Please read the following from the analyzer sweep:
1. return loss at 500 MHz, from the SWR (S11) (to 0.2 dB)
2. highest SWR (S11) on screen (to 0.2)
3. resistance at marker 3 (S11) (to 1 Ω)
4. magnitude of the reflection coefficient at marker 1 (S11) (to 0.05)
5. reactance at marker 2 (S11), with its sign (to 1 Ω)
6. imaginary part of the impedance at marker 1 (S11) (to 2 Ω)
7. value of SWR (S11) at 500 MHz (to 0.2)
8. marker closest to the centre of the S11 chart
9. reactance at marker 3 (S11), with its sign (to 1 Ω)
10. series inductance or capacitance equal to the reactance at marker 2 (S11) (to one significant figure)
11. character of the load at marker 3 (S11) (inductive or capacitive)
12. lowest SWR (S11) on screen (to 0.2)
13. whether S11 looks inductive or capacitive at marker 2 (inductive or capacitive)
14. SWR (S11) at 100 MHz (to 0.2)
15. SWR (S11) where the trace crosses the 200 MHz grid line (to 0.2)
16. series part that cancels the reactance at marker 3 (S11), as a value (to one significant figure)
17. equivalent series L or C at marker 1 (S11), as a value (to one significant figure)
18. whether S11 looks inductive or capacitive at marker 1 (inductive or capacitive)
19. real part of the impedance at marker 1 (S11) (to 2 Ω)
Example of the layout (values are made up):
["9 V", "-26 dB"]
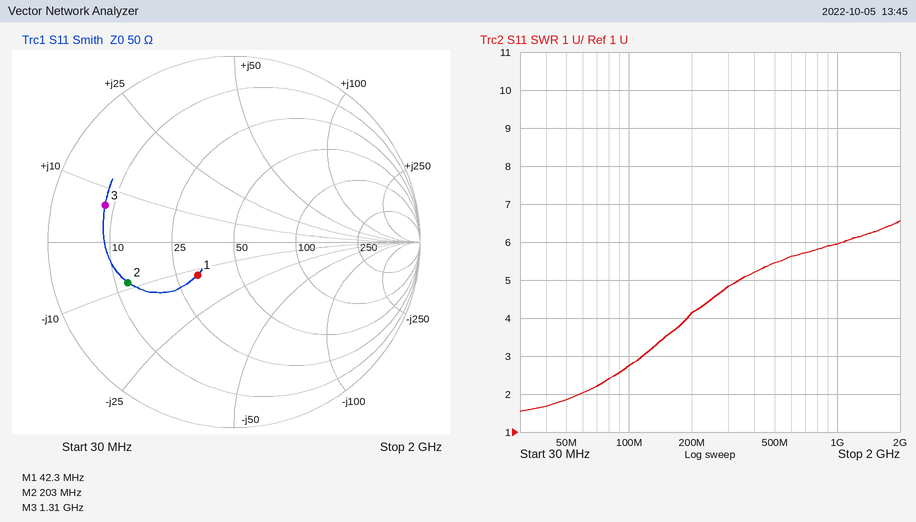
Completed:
["3.2 dB", "6.6", "8 Ω", "0.25", "-9 Ω", "-12 Ω", "5.4", "marker 1", "+7 Ω", "90 pF", "inductive", "1.6", "capacitive", "2.8", "4.2", "20 pF", "300 pF", "capacitive", "32 Ω"]
